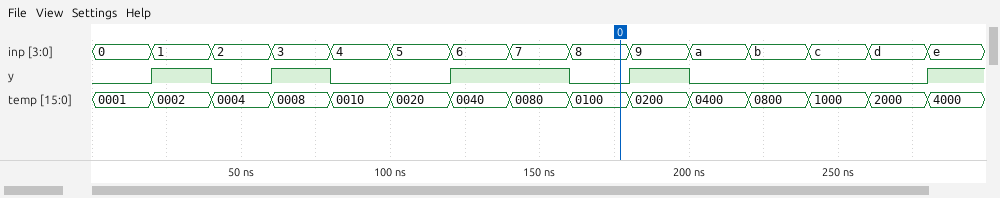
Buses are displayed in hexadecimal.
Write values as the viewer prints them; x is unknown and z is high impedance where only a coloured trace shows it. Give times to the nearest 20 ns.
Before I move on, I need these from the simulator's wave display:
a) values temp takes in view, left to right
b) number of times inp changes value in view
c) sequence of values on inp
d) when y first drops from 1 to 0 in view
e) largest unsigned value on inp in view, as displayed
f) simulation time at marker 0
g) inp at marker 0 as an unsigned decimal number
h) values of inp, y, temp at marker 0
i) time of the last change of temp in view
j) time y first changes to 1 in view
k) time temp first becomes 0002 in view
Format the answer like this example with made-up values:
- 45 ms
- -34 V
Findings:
- 0001, 0002, 0004, 0008, 0010, 0020, 0040, 0080, 0100, 0200, 0400, 0800, 1000, 2000, 4000
- 14
- 0, 1, 2, 3, 4, 5, 6, 7, 8, 9, a, b, c, d, e
- 40 ns
- e
- 180 ns
- 8
- inp=8, y=0, temp=0100
- 280 ns
- 20 ns
- 20 ns
